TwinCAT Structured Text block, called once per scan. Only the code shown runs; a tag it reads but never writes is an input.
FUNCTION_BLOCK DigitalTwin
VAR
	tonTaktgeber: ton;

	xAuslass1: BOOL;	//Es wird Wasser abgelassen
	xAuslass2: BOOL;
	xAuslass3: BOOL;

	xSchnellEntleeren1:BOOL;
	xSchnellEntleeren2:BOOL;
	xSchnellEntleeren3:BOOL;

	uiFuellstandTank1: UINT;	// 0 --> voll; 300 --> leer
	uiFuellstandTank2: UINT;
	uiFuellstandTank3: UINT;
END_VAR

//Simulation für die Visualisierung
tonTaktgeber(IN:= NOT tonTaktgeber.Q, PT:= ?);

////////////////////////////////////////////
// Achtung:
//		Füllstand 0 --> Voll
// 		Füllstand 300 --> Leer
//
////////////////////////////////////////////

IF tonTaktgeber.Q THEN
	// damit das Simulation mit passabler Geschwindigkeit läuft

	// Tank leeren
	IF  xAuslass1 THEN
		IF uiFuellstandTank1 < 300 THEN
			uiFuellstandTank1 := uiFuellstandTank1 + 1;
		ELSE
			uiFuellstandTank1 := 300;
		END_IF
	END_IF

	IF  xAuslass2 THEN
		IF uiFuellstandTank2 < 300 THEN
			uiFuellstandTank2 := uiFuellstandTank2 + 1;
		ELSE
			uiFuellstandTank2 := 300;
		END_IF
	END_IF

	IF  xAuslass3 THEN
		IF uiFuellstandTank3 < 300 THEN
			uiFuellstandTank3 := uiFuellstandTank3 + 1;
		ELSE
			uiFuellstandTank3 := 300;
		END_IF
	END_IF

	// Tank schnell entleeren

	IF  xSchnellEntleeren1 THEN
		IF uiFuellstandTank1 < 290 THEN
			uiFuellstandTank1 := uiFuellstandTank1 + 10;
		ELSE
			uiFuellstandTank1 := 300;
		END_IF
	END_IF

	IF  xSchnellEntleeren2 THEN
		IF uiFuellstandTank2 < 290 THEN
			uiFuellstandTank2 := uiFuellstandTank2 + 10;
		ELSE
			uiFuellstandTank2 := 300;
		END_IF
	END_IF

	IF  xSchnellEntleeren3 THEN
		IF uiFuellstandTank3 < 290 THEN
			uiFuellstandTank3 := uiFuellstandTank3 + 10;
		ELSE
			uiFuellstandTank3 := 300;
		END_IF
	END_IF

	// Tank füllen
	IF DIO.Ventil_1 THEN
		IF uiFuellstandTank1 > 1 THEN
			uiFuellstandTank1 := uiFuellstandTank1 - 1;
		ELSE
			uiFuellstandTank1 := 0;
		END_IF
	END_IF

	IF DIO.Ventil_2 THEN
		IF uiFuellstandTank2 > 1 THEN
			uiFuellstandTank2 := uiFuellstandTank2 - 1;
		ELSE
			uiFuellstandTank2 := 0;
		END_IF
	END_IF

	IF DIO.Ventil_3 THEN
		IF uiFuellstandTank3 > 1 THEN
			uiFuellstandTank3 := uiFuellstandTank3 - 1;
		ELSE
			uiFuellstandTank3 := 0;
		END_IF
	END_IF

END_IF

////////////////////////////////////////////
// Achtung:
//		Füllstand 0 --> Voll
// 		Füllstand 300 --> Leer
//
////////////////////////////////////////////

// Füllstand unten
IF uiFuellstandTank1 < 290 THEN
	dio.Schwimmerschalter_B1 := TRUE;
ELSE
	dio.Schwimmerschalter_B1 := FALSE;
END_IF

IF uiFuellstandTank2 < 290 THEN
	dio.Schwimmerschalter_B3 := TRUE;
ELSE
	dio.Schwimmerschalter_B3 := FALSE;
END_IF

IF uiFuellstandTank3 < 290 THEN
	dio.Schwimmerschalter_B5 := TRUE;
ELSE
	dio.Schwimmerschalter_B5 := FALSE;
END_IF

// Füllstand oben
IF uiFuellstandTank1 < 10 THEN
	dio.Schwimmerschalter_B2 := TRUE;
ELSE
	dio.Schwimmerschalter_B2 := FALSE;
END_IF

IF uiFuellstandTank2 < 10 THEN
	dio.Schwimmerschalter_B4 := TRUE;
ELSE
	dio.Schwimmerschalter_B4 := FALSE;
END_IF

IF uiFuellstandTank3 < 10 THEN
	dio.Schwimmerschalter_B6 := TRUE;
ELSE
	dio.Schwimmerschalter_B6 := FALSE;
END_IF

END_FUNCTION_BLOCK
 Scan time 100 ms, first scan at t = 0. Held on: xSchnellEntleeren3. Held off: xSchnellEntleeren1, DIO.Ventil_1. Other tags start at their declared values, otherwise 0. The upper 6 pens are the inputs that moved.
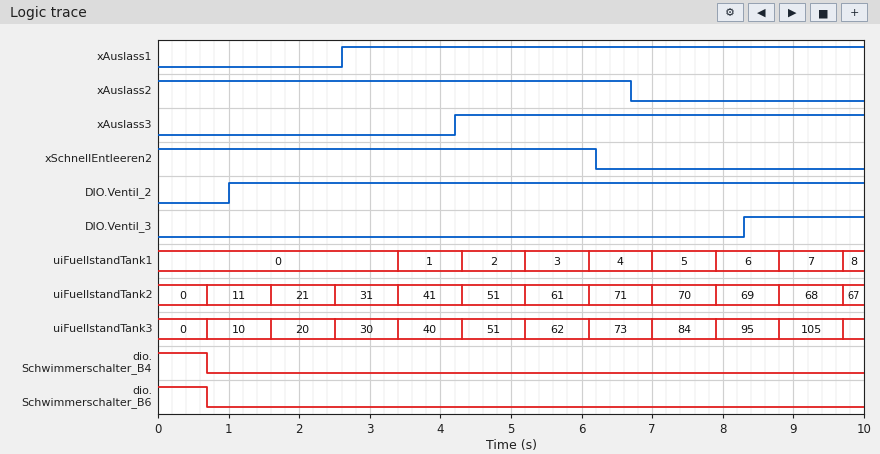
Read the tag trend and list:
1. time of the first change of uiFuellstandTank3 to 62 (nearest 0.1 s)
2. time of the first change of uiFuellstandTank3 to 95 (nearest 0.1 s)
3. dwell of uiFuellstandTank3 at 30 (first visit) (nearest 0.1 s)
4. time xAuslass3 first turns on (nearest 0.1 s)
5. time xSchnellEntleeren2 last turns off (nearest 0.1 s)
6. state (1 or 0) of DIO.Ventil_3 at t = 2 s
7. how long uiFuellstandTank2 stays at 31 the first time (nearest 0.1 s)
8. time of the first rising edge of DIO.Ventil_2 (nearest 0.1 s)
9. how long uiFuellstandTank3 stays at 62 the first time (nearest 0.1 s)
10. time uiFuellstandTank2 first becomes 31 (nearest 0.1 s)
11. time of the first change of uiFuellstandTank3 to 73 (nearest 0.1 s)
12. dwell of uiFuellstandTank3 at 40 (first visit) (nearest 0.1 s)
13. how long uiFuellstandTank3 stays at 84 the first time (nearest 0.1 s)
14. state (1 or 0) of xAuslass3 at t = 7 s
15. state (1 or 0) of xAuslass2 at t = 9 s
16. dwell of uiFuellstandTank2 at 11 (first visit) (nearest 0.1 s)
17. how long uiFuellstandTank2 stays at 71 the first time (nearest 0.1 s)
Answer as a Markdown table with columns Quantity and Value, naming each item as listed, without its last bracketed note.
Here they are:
| Quantity | Value |
|---|---|
| time of the first change of uiFuellstandTank3 to 62 | 5.2 s |
| time of the first change of uiFuellstandTank3 to 95 | 7.9 s |
| dwell of uiFuellstandTank3 at 30 (first visit) | 0.9 s |
| time xAuslass3 first turns on | 4.2 s |
| time xSchnellEntleeren2 last turns off | 6.2 s |
| state (1 or 0) of DIO.Ventil_3 at t = 2 s | 0 |
| how long uiFuellstandTank2 stays at 31 the first time | 0.9 s |
| time of the first rising edge of DIO.Ventil_2 | 1.0 s |
| how long uiFuellstandTank3 stays at 62 the first time | 0.9 s |
| time uiFuellstandTank2 first becomes 31 | 2.5 s |
| time of the first change of uiFuellstandTank3 to 73 | 6.1 s |
| dwell of uiFuellstandTank3 at 40 (first visit) | 0.9 s |
| how long uiFuellstandTank3 stays at 84 the first time | 0.9 s |
| state (1 or 0) of xAuslass3 at t = 7 s | 1 |
| state (1 or 0) of xAuslass2 at t = 9 s | 0 |
| dwell of uiFuellstandTank2 at 11 (first visit) | 0.9 s |
| how long uiFuellstandTank2 stays at 71 the first time | 0.9 s |
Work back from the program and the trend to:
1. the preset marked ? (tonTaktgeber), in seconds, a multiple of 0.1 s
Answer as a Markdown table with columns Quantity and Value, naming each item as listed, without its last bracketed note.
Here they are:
| Quantity | Value |
|---|---|
| the preset marked ? (tonTaktgeber), in seconds, a multiple of 0.1 s | 0.7 s |
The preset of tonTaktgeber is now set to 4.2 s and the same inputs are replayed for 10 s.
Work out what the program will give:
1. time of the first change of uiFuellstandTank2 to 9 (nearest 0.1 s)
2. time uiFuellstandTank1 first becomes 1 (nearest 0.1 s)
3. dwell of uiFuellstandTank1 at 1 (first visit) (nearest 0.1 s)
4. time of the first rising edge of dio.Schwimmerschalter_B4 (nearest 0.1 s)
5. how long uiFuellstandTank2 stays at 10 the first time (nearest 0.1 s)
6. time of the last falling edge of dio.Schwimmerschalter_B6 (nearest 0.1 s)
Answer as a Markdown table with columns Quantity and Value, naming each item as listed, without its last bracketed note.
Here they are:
| Quantity | Value |
|---|---|
| time of the first change of uiFuellstandTank2 to 9 | 8.6 s |
| time uiFuellstandTank1 first becomes 1 | 4.2 s |
| dwell of uiFuellstandTank1 at 1 (first visit) | 4.4 s |
| time of the first rising edge of dio.Schwimmerschalter_B4 | 8.6 s |
| how long uiFuellstandTank2 stays at 10 the first time | 4.4 s |
| time of the last falling edge of dio.Schwimmerschalter_B6 | 4.2 s |
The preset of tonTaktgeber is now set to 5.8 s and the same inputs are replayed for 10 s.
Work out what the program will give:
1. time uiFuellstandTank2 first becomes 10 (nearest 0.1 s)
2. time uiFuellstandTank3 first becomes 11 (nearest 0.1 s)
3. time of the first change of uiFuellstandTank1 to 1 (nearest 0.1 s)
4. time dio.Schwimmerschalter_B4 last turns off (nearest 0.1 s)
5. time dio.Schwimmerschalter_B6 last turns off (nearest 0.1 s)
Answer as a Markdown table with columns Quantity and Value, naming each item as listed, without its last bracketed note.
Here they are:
| Quantity | Value |
|---|---|
| time uiFuellstandTank2 first becomes 10 | 5.8 s |
| time uiFuellstandTank3 first becomes 11 | 5.8 s |
| time of the first change of uiFuellstandTank1 to 1 | 5.8 s |
| time dio.Schwimmerschalter_B4 last turns off | 5.8 s |
| time dio.Schwimmerschalter_B6 last turns off | 5.8 s |
